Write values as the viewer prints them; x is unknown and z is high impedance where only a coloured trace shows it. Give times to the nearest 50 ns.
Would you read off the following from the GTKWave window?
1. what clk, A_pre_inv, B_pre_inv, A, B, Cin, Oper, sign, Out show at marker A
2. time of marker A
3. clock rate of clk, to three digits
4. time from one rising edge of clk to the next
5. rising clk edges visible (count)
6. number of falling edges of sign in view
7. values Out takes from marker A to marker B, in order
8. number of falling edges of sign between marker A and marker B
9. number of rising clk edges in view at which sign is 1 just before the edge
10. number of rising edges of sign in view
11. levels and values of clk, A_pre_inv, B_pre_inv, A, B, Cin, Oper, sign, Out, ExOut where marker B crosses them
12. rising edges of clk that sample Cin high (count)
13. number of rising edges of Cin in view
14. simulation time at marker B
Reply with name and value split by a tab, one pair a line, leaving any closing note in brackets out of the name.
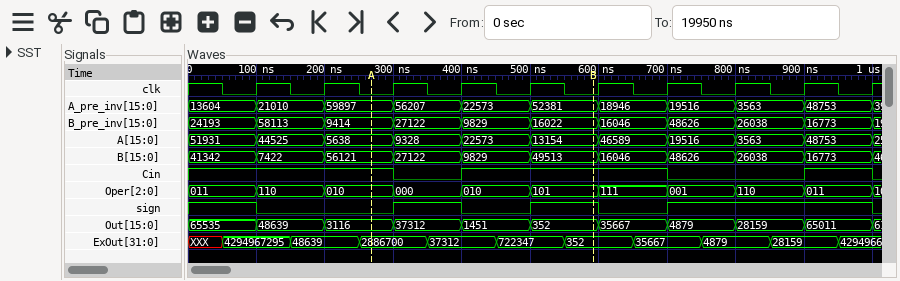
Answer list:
what clk, A_pre_inv, B_pre_inv, A, B, Cin, Oper, sign, Out show at marker A	clk=0, A_pre_inv=59897, B_pre_inv=9414, A=5638, B=56121, Cin=1, Oper=010, sign=0, Out=3116
time of marker A	250 ns
clock rate of clk, to three digits	10.0 MHz
time from one rising edge of clk to the next	100 ns
rising clk edges visible	10
number of falling edges of sign in view	4
values Out takes from marker A to marker B, in order	3116, 37312, 1451, 352
number of falling edges of sign between marker A and marker B	1
number of rising clk edges in view at which sign is 1 just before the edge	6
number of rising edges of sign in view	3
levels and values of clk, A_pre_inv, B_pre_inv, A, B, Cin, Oper, sign, Out, ExOut where marker B crosses them	clk=0, A_pre_inv=52381, B_pre_inv=16022, A=13154, B=49513, Cin=1, Oper=101, sign=1, Out=352, ExOut=352
rising edges of clk that sample Cin high	7
number of rising edges of Cin in view	2
simulation time at marker B	600 ns
